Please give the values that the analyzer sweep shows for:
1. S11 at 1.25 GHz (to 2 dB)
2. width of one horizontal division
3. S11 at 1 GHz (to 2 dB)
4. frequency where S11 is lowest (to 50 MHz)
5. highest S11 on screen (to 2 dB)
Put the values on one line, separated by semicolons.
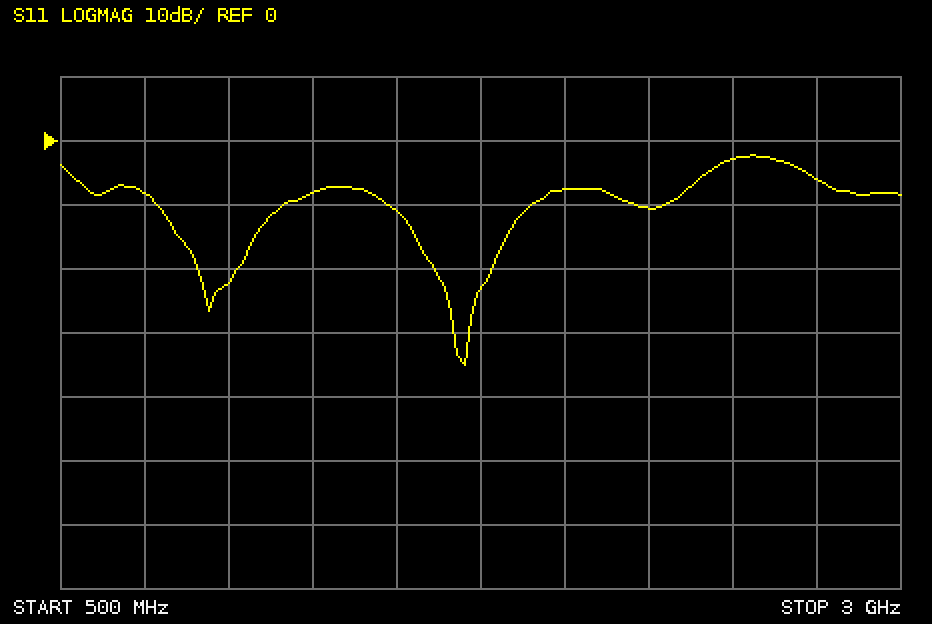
-8 dB; 250 MHz; -22 dB; 1.70 GHz; -2 dB
